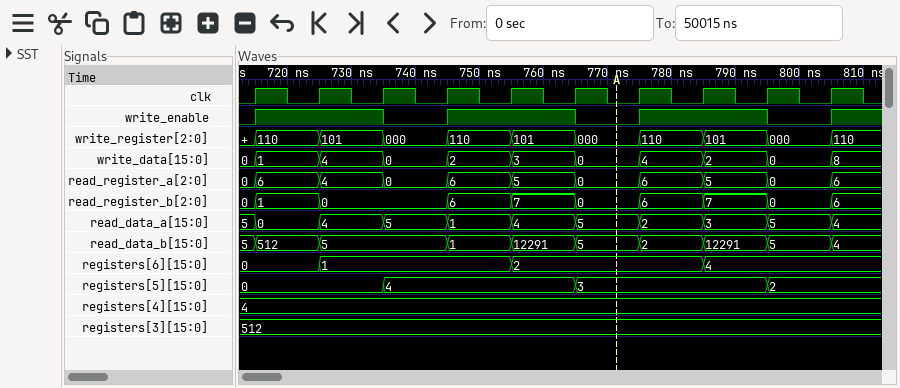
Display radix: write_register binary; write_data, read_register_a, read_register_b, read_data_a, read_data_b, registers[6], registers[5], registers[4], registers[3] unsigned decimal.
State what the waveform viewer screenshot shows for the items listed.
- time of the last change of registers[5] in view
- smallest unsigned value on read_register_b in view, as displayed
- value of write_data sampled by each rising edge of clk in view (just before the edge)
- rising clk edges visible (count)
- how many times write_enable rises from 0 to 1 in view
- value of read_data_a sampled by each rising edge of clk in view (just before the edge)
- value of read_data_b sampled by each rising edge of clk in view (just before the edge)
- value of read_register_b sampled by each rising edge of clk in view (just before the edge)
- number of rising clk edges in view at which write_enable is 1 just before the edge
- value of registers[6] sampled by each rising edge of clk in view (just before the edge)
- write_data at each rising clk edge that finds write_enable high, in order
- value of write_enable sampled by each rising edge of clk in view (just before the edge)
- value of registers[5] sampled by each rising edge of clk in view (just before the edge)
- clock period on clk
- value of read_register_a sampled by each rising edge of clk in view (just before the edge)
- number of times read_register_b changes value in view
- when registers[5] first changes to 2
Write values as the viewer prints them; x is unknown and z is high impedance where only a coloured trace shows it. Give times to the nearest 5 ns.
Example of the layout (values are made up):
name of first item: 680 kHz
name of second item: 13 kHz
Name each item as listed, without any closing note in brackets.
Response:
time of the last change of registers[5] in view: 795 ns
smallest unsigned value on read_register_b in view, as displayed: 0
value of write_data sampled by each rising edge of clk in view: 0, 1, 4, 0, 2, 3, 0, 4, 2, 0
rising clk edges visible: 10
how many times write_enable rises from 0 to 1 in view: 4
value of read_data_a sampled by each rising edge of clk in view: 5, 0, 4, 5, 1, 4, 5, 2, 3, 5
value of read_data_b sampled by each rising edge of clk in view: 5, 512, 5, 5, 1, 12291, 5, 2, 12291, 5
value of read_register_b sampled by each rising edge of clk in view: 0, 1, 0, 0, 6, 7, 0, 6, 7, 0
number of rising clk edges in view at which write_enable is 1 just before the edge: 6
value of registers[6] sampled by each rising edge of clk in view: 0, 0, 1, 1, 1, 2, 2, 2, 4, 4
write_data at each rising clk edge that finds write_enable high, in order: 1, 4, 2, 3, 4, 2
value of write_enable sampled by each rising edge of clk in view: 0 1 1 0 1 1 0 1 1 0
value of registers[5] sampled by each rising edge of clk in view: 0, 0, 0, 4, 4, 4, 3, 3, 3, 2
clock period on clk: 10 ns
value of read_register_a sampled by each rising edge of clk in view: 0, 6, 4, 0, 6, 5, 0, 6, 5, 0
number of times read_register_b changes value in view: 9
when registers[5] first changes to 2: 795 ns
